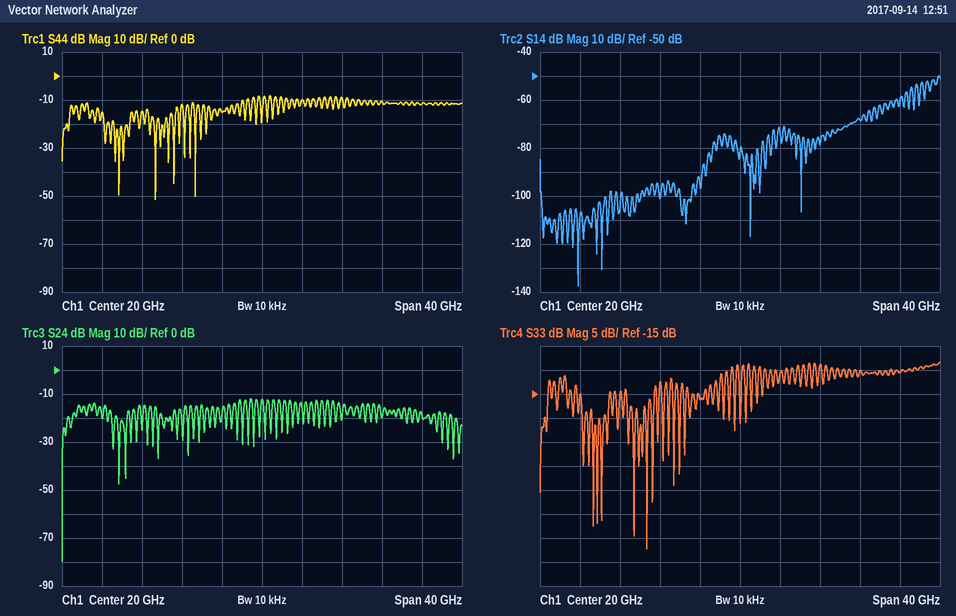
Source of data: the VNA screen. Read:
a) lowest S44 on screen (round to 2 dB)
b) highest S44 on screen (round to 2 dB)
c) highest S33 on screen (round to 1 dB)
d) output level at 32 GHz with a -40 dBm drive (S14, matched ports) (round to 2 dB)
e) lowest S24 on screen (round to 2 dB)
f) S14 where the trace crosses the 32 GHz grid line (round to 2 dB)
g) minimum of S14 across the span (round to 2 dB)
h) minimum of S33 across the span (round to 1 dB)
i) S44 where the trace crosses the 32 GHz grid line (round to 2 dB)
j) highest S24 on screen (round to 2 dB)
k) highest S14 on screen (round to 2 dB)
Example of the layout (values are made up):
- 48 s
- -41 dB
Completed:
- -52 dB
- -8 dB
- -8 dB
- -108 dBm
- -80 dB
- -68 dB
- -138 dB
- -47 dB
- -10 dB
- -12 dB
- -50 dB
